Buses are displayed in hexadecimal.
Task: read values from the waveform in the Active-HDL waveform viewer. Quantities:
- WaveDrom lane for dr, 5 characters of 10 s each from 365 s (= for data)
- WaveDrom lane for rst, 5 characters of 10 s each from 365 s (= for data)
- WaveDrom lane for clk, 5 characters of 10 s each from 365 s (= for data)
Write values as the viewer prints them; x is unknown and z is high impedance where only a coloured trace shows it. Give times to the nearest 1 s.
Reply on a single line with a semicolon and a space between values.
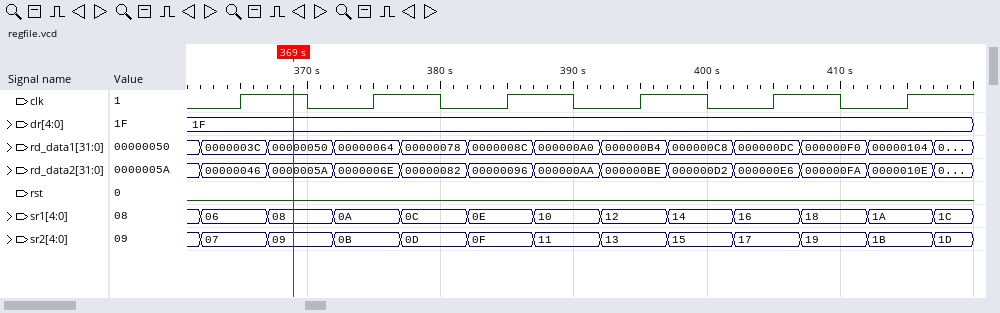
{name: 'dr', wave: '=....', data: '1F'}; {name: 'rst', wave: '0....'}; {name: 'clk', wave: 'p....'}
